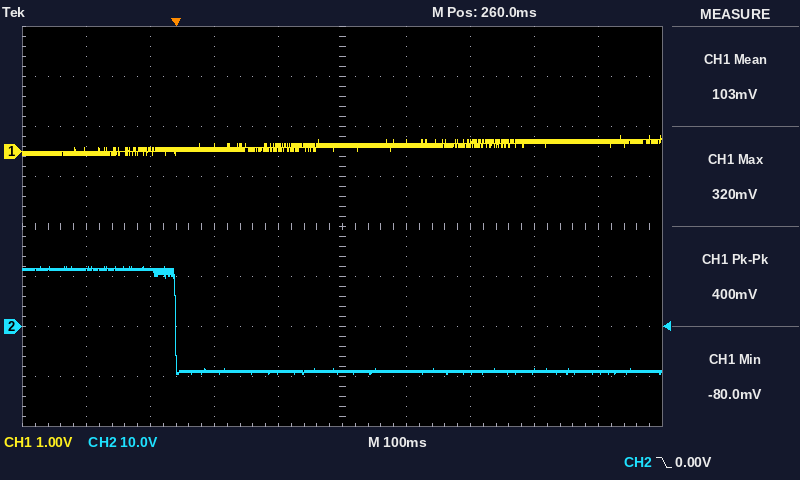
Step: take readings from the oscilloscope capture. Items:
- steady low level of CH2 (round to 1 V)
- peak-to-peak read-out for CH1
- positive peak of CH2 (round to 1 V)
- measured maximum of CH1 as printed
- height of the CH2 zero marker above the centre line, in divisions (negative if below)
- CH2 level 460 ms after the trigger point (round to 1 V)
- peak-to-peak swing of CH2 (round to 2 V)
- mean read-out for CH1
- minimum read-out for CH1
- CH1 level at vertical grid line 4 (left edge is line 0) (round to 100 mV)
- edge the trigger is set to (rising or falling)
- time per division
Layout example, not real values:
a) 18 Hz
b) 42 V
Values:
a) -9 V
b) 400 mV
c) 12 V
d) 320 mV
e) -2.0 div
f) -9 V
g) 22 V
h) 103 mV
i) -80.0 mV
j) 100 mV
k) falling
l) 100 ms
